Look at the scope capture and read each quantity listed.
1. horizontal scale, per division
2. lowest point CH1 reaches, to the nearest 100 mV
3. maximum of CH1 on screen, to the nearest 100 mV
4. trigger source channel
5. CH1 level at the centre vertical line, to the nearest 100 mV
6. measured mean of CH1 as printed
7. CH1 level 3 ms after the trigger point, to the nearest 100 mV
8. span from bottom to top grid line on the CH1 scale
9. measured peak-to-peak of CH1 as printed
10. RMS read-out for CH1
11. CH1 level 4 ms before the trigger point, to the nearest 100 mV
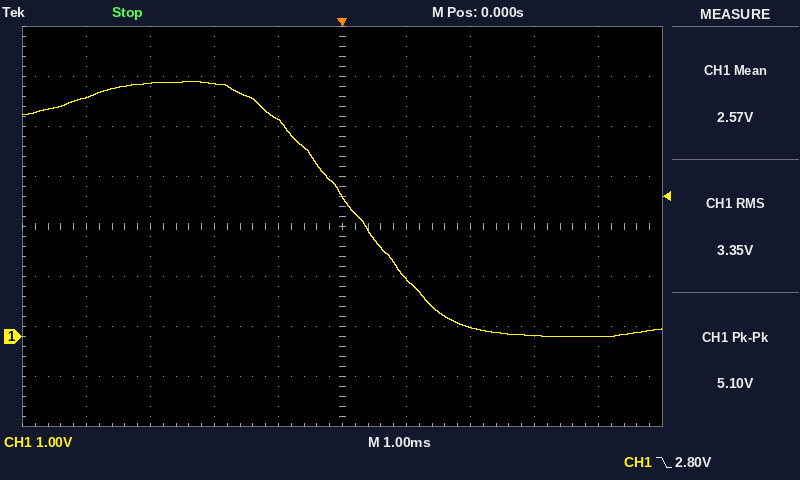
1 ms
0.0 V
5.1 V
CH1
2.8 V
2.57 V
0.0 V
8 V
5.10 V
3.35 V
4.8 V
